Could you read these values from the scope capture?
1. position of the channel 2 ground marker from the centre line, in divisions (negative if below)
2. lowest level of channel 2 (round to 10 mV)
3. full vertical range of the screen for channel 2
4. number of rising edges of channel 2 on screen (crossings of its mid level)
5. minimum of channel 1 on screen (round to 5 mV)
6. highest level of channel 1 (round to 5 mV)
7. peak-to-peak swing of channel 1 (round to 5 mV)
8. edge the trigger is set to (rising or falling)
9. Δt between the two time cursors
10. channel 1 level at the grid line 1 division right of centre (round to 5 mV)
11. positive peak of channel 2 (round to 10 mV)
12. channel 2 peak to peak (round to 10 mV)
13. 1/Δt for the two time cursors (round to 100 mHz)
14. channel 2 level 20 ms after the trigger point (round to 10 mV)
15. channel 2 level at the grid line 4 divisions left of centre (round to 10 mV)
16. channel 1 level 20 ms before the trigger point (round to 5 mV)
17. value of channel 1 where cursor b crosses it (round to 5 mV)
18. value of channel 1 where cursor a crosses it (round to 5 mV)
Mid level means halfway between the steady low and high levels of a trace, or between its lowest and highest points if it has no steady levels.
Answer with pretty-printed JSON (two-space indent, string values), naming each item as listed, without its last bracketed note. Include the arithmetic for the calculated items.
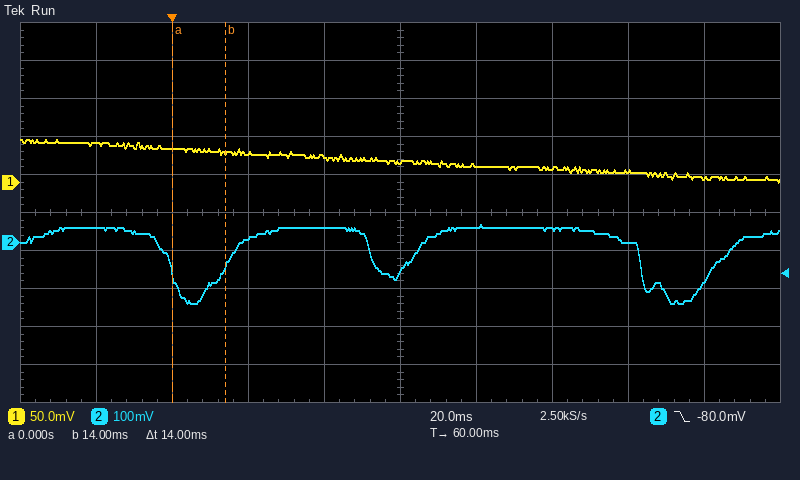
{
  "position of the channel 2 ground marker from the centre line, in divisions": "-0.8 div",
  "lowest level of channel 2": "-160 mV",
  "full vertical range of the screen for channel 2": "1 V",
  "number of rising edges of channel 2 on screen": "3",
  "minimum of channel 1 on screen": "0 mV",
  "highest level of channel 1": "55 mV",
  "peak-to-peak swing of channel 1": "55 mV − (0 mV) = 55 mV",
  "edge the trigger is set to": "falling",
  "Δt between the two time cursors": "14 ms",
  "channel 1 level at the grid line 1 division right of centre": "20 mV",
  "positive peak of channel 2": "50 mV",
  "channel 2 peak to peak": "50 mV − (-160 mV) = 210 mV",
  "1/Δt for the two time cursors": "1 / 14 ms ≈ 71.4 Hz",
  "channel 2 level 20 ms after the trigger point": "10 mV",
  "channel 2 level at the grid line 4 divisions left of centre": "40 mV",
  "channel 1 level 20 ms before the trigger point": "50 mV",
  "value of channel 1 where cursor b crosses it": "40 mV",
  "value of channel 1 where cursor a crosses it": "45 mV"
}
